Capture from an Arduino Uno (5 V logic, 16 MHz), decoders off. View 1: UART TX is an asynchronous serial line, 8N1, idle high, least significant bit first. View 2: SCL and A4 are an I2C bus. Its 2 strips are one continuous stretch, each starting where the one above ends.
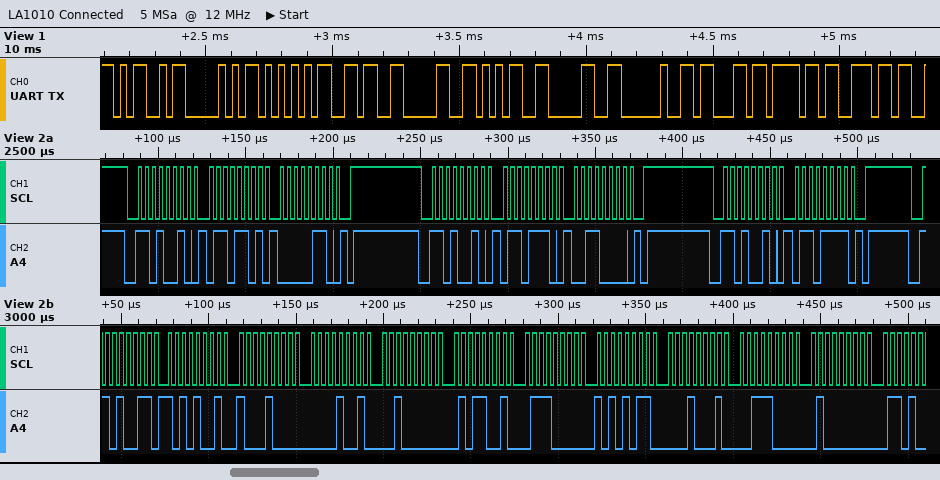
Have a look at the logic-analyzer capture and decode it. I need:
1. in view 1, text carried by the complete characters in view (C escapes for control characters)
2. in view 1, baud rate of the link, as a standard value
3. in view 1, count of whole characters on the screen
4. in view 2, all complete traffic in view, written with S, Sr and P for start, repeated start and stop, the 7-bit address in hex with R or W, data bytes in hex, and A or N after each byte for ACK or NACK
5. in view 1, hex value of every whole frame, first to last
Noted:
"MPU6050 con"
38400 baud
11
S 69W A 6D A 06 A P S 69W A 6E A 30 A P S 69W A 6F A P S 69R A A9 A 88 A 09 A 20 A 59 A 70 A AB A 11 A 38 A 40 A
4D 50 55 36 30 35 30 20 63 6F 6E
